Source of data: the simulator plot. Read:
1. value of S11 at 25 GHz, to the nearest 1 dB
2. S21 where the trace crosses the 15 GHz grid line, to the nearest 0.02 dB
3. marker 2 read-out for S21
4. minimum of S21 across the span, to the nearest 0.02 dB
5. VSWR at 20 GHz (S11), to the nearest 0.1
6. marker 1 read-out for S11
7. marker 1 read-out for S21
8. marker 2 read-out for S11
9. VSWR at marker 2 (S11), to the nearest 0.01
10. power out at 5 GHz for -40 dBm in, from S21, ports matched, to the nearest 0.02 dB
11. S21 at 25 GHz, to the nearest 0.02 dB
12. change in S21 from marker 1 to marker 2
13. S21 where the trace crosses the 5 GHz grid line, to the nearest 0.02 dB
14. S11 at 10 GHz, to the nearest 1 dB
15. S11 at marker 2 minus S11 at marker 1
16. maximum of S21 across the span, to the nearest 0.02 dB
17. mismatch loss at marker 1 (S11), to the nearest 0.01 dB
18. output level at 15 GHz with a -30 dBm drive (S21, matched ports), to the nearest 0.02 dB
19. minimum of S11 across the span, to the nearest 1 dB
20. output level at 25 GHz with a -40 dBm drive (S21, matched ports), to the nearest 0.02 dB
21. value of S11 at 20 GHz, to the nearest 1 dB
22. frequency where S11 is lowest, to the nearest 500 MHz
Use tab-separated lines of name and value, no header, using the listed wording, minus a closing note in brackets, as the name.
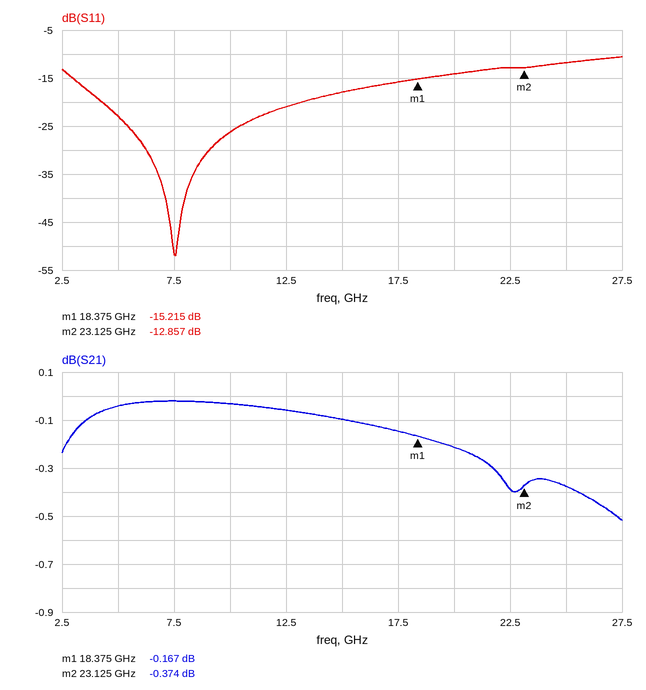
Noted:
value of S11 at 25 GHz, to the nearest 1 dB	-12 dB
S21 where the trace crosses the 15 GHz grid line, to the nearest 0.02 dB	-0.10 dB
marker 2 read-out for S21	-0.374 dB
minimum of S21 across the span, to the nearest 0.02 dB	-0.52 dB
VSWR at 20 GHz (S11), to the nearest 0.1	1.5
marker 1 read-out for S11	-15.215 dB
marker 1 read-out for S21	-0.167 dB
marker 2 read-out for S11	-12.857 dB
VSWR at marker 2 (S11), to the nearest 0.01	1.59
power out at 5 GHz for -40 dBm in, from S21, ports matched, to the nearest 0.02 dB	-40.04 dBm
S21 at 25 GHz, to the nearest 0.02 dB	-0.38 dB
change in S21 from marker 1 to marker 2	-0.207 dB
S21 where the trace crosses the 5 GHz grid line, to the nearest 0.02 dB	-0.04 dB
S11 at 10 GHz, to the nearest 1 dB	-26 dB
S11 at marker 2 minus S11 at marker 1	2.358 dB
maximum of S21 across the span, to the nearest 0.02 dB	-0.02 dB
mismatch loss at marker 1 (S11), to the nearest 0.01 dB	0.13 dB
output level at 15 GHz with a -30 dBm drive (S21, matched ports), to the nearest 0.02 dB	-30.10 dBm
minimum of S11 across the span, to the nearest 1 dB	-52 dB
output level at 25 GHz with a -40 dBm drive (S21, matched ports), to the nearest 0.02 dB	-40.38 dBm
value of S11 at 20 GHz, to the nearest 1 dB	-14 dB
frequency where S11 is lowest, to the nearest 500 MHz	7.5 GHz
